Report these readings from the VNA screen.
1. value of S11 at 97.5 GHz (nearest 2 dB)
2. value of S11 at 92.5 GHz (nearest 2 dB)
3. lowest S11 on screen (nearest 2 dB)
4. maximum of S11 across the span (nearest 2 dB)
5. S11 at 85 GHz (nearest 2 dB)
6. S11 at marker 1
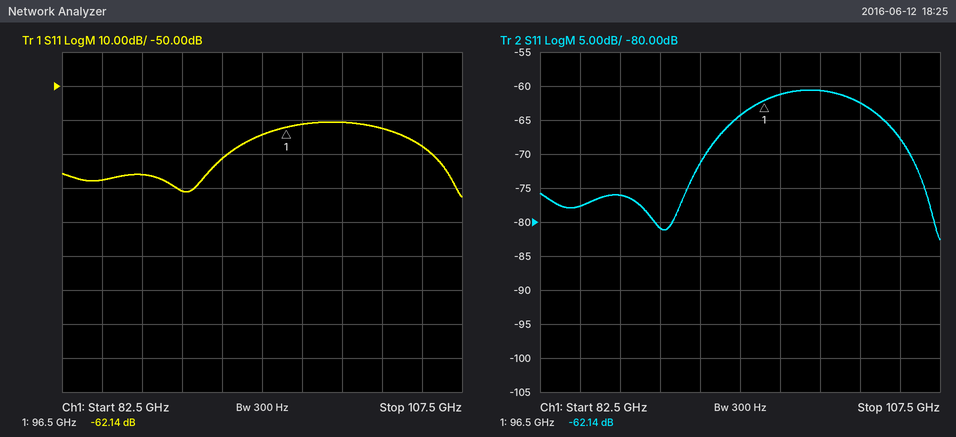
-62 dB
-72 dB
-82 dB
-60 dB
-78 dB
-62.14 dB
